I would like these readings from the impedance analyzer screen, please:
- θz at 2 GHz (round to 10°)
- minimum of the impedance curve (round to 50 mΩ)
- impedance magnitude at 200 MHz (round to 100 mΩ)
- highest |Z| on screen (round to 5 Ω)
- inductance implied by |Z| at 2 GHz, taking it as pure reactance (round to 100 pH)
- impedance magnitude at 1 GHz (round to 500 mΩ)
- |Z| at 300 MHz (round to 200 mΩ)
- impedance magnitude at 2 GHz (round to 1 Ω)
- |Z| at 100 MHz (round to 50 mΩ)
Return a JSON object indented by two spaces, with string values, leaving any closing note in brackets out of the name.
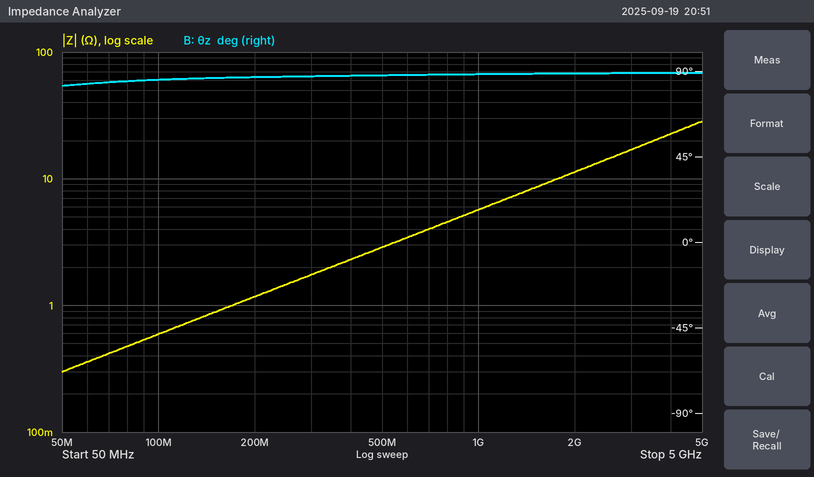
{
  "θz at 2 GHz": "90°",
  "minimum of the impedance curve": "300 mΩ",
  "impedance magnitude at 200 MHz": "1.2 Ω",
  "highest |Z| on screen": "30 Ω",
  "inductance implied by |Z| at 2 GHz, taking it as pure reactance": "900 pH",
  "impedance magnitude at 1 GHz": "5.5 Ω",
  "|Z| at 300 MHz": "1.8 Ω",
  "impedance magnitude at 2 GHz": "11 Ω",
  "|Z| at 100 MHz": "600 mΩ"
}
